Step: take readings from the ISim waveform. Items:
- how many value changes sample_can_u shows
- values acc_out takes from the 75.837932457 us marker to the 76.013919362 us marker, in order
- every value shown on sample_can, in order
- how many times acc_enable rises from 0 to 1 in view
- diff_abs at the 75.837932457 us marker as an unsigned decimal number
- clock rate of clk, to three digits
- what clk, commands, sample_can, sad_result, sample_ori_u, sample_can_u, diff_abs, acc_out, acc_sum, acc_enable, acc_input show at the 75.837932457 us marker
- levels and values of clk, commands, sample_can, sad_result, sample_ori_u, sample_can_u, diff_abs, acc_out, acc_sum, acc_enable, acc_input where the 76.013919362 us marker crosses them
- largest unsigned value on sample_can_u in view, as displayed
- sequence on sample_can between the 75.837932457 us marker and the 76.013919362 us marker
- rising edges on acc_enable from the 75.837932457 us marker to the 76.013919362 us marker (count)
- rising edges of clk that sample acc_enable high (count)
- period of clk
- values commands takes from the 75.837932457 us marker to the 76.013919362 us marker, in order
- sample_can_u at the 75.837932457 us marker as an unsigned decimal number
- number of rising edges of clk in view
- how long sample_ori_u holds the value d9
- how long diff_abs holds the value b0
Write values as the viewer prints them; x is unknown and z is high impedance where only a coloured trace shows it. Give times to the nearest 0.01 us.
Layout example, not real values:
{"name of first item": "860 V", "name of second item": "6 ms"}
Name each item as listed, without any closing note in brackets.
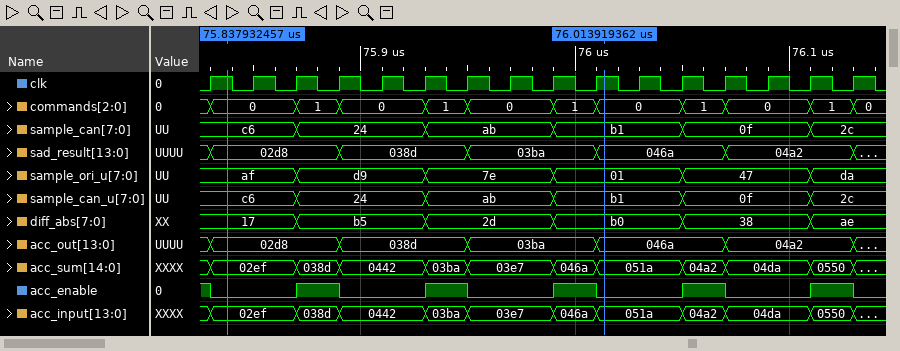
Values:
{"how many value changes sample_can_u shows": "5", "values acc_out takes from the 75.837932457 us marker to the 76.013919362 us marker, in order": "02d8, 038d, 03ba, 046a", "every value shown on sample_can, in order": "c6, 24, ab, b1, 0f, 2c", "how many times acc_enable rises from 0 to 1 in view": "5", "diff_abs at the 75.837932457 us marker as an unsigned decimal number": "23", "clock rate of clk, to three digits": "50.0 MHz", "what clk, commands, sample_can, sad_result, sample_ori_u, sample_can_u, diff_abs, acc_out, acc_sum, acc_enable, acc_input show at the 75.837932457 us marker": "clk=1, commands=0, sample_can=c6, sad_result=02d8, sample_ori_u=af, sample_can_u=c6, diff_abs=17, acc_out=02d8, acc_sum=02ef, acc_enable=0, acc_input=02ef", "levels and values of clk, commands, sample_can, sad_result, sample_ori_u, sample_can_u, diff_abs, acc_out, acc_sum, acc_enable, acc_input where the 76.013919362 us marker crosses them": "clk=1, commands=0, sample_can=b1, sad_result=046a, sample_ori_u=01, sample_can_u=b1, diff_abs=b0, acc_out=046a, acc_sum=051a, acc_enable=0, acc_input=051a", "largest unsigned value on sample_can_u in view, as displayed": "c6", "sequence on sample_can between the 75.837932457 us marker and the 76.013919362 us marker": "c6, 24, ab, b1", "rising edges on acc_enable from the 75.837932457 us marker to the 76.013919362 us marker": "3", "rising edges of clk that sample acc_enable high": "6", "period of clk": "0.02 us", "values commands takes from the 75.837932457 us marker to the 76.013919362 us marker, in order": "0, 1, 0, 1, 0, 1, 0", "sample_can_u at the 75.837932457 us marker as an unsigned decimal number": "198", "number of rising edges of clk in view": "16", "how long sample_ori_u holds the value d9": "0.06 us", "how long diff_abs holds the value b0": "0.06 us"}
